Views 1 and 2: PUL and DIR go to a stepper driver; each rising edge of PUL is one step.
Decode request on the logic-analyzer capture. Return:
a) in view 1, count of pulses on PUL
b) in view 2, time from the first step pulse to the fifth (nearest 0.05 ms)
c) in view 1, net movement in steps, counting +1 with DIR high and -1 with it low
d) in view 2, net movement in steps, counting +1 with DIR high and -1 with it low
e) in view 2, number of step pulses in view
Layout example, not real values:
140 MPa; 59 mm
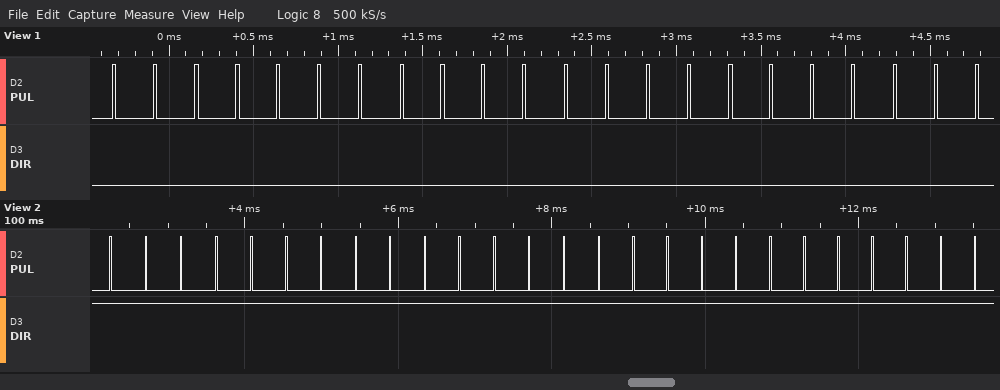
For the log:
22; 1.85 ms; -22; +26; 26
